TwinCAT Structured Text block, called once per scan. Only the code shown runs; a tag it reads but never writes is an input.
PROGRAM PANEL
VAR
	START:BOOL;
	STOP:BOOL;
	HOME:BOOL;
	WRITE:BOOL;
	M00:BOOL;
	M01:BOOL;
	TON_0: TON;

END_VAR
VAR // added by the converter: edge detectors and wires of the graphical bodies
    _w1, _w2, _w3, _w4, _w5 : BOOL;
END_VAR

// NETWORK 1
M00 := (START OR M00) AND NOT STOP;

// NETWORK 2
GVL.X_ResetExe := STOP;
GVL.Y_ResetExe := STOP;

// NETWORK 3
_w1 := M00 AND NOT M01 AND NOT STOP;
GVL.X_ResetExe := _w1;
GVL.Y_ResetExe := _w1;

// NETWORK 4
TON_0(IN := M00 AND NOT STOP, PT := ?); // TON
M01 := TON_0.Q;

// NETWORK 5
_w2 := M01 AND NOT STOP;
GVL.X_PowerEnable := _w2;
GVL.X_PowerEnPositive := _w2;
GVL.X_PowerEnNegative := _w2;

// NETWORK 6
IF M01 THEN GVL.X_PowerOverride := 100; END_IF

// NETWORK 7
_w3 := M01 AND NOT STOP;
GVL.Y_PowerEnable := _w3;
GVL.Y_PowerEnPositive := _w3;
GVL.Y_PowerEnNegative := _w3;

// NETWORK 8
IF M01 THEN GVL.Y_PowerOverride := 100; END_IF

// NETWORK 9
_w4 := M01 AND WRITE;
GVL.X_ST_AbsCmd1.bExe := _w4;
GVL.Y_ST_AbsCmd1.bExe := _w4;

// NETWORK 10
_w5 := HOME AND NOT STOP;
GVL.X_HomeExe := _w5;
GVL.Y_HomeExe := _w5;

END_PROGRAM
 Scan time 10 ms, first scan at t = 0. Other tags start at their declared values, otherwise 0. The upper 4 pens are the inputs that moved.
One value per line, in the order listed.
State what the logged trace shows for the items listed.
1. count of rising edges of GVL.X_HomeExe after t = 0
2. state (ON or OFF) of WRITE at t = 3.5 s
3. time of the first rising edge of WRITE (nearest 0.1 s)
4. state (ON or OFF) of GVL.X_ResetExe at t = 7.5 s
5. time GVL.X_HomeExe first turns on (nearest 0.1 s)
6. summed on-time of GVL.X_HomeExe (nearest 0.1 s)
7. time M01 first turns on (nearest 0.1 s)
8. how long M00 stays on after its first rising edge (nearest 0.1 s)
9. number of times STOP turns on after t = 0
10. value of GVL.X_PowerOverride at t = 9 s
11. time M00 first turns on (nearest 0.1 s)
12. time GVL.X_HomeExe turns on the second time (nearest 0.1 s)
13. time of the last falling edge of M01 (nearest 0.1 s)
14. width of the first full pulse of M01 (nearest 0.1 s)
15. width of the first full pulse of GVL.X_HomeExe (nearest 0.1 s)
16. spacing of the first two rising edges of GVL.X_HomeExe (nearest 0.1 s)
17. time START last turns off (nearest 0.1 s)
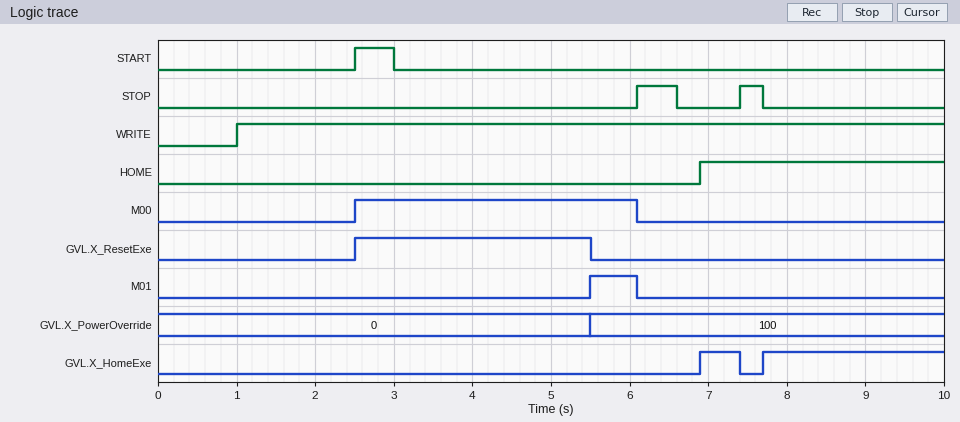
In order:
2
ON
1.0 s
OFF
6.9 s
2.8 s
5.5 s
3.6 s
2
100
2.5 s
7.7 s
6.1 s
0.6 s
0.5 s
0.8 s
3.0 s
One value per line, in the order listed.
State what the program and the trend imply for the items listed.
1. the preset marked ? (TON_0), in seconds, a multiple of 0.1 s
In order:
3.0 s
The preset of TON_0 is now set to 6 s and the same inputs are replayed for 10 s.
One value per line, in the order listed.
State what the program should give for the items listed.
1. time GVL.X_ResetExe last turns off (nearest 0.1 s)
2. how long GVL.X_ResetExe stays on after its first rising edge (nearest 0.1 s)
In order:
6.1 s
3.6 s
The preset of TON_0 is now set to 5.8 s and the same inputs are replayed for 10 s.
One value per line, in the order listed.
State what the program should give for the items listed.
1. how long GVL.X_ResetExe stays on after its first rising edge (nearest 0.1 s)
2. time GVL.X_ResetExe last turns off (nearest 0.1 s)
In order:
3.6 s
6.1 s
